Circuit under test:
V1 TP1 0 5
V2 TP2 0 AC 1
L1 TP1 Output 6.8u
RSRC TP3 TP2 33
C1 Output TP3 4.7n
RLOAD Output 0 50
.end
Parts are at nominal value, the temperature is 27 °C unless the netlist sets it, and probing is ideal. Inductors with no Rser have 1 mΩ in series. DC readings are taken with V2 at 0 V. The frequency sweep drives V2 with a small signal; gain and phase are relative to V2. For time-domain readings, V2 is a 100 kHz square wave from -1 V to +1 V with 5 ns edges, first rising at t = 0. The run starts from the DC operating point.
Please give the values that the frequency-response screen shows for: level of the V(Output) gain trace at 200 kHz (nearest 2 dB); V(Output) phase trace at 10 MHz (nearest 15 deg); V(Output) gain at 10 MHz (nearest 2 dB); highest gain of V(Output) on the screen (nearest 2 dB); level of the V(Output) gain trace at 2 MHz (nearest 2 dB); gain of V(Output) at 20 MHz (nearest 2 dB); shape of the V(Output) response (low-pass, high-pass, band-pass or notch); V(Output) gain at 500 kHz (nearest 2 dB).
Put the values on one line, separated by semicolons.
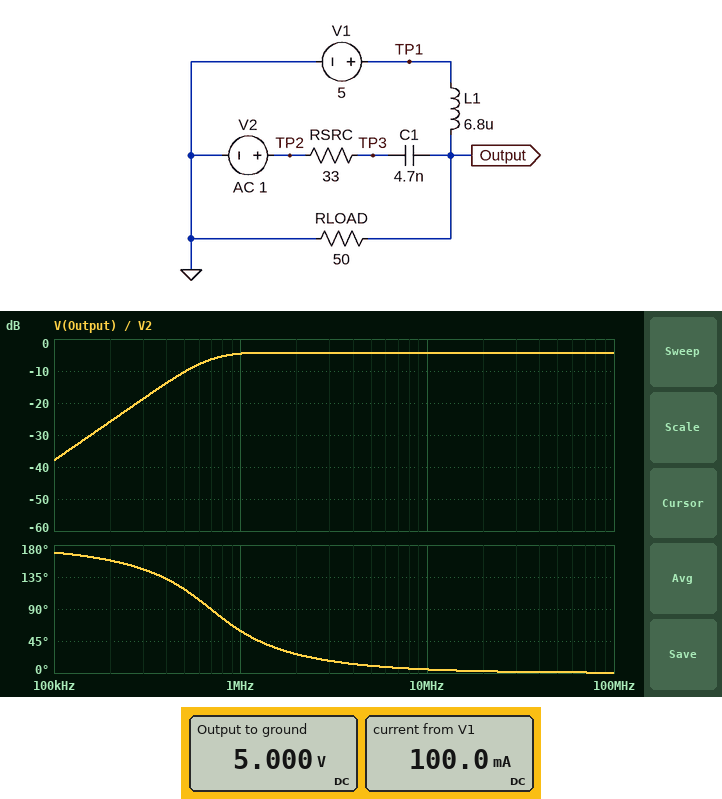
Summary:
-26 dB; 0 deg; -4 dB; -4 dB; -4 dB; -4 dB; high-pass; -10 dB
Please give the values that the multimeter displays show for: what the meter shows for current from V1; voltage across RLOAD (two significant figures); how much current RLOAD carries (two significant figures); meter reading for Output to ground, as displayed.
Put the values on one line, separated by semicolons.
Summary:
100.0 mA; 5.0 V; 100 mA; 5.000 V
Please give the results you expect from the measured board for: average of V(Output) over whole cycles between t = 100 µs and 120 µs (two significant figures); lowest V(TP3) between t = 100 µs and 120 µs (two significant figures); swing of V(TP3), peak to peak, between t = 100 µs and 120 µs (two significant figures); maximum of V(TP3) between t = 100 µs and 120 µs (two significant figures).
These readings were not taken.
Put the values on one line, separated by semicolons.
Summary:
5.0 V; -1.1 V; 2.1 V; 1.1 V
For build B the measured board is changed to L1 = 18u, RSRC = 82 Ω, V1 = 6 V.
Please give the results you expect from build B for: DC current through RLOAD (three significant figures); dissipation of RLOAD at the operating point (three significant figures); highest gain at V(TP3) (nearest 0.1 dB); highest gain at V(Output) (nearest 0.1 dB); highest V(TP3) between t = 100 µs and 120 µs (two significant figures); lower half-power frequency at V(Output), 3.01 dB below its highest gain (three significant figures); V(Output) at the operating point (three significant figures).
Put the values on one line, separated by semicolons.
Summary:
120 mA; 720 mW; 0 dB; -8.4 dB; 1.0 V; 380 kHz; 6.00 V
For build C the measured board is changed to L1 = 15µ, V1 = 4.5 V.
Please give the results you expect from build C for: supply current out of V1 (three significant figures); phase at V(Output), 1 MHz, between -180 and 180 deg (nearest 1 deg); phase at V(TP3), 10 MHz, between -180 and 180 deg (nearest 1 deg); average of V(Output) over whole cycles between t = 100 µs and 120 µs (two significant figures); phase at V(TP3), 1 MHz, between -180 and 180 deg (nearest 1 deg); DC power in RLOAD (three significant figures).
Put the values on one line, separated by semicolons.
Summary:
90.0 mA; 38 deg; 0 deg; 4.5 V; -8 deg; 405 mW
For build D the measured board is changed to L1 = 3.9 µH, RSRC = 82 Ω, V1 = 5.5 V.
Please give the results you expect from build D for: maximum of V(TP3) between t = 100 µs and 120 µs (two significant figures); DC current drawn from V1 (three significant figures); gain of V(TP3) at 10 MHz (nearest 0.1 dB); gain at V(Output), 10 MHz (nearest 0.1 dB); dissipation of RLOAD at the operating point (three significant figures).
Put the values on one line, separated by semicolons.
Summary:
1.0 V; 110 mA; -8.6 dB; -8.5 dB; 605 mW
